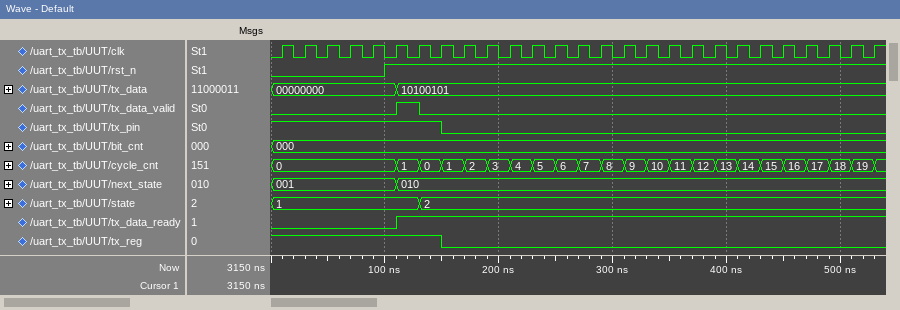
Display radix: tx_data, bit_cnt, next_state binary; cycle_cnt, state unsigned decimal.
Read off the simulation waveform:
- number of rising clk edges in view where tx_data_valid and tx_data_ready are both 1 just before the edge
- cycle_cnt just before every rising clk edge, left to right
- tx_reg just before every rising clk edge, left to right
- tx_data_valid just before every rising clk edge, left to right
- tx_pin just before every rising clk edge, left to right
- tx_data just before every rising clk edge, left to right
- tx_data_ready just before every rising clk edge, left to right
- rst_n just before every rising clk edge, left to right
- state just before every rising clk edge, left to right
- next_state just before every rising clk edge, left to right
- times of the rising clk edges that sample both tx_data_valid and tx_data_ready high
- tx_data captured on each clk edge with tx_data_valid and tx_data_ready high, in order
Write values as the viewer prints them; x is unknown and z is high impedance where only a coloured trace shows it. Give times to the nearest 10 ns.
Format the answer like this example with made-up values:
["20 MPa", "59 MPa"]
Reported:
["1", "0, 0, 0, 0, 0, 0, 1, 0, 1, 2, 3, 4, 5, 6, 7, 8, 9, 10, 11, 12, 13, 14, 15, 16, 17, 18, 19", "1 1 1 1 1 1 1 1 0 0 0 0 0 0 0 0 0 0 0 0 0 0 0 0 0 0 0", "0 0 0 0 0 0 1 0 0 0 0 0 0 0 0 0 0 0 0 0 0 0 0 0 0 0 0", "1 1 1 1 1 1 1 1 0 0 0 0 0 0 0 0 0 0 0 0 0 0 0 0 0 0 0", "00000000, 00000000, 00000000, 00000000, 00000000, 00000000, 10100101, 10100101, 10100101, 10100101, 10100101, 10100101, 10100101, 10100101, 10100101, 10100101, 10100101, 10100101, 10100101, 10100101, 10100101, 10100101, 10100101, 10100101, 10100101, 10100101, 10100101", "0 0 0 0 0 0 1 1 1 1 1 1 1 1 1 1 1 1 1 1 1 1 1 1 1 1 1", "0 0 0 0 0 1 1 1 1 1 1 1 1 1 1 1 1 1 1 1 1 1 1 1 1 1 1", "1, 1, 1, 1, 1, 1, 1, 2, 2, 2, 2, 2, 2, 2, 2, 2, 2, 2, 2, 2, 2, 2, 2, 2, 2, 2, 2", "001, 001, 001, 001, 001, 001, 010, 010, 010, 010, 010, 010, 010, 010, 010, 010, 010, 010, 010, 010, 010, 010, 010, 010, 010, 010, 010", "130 ns", "10100101"]
